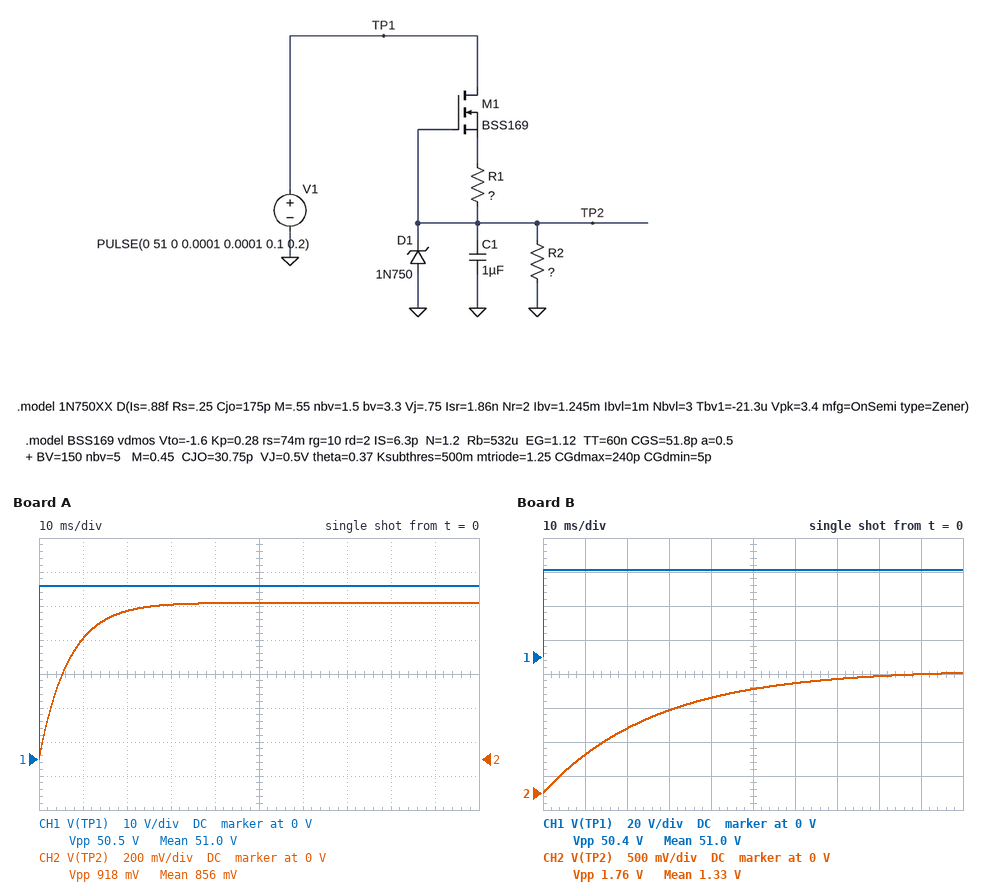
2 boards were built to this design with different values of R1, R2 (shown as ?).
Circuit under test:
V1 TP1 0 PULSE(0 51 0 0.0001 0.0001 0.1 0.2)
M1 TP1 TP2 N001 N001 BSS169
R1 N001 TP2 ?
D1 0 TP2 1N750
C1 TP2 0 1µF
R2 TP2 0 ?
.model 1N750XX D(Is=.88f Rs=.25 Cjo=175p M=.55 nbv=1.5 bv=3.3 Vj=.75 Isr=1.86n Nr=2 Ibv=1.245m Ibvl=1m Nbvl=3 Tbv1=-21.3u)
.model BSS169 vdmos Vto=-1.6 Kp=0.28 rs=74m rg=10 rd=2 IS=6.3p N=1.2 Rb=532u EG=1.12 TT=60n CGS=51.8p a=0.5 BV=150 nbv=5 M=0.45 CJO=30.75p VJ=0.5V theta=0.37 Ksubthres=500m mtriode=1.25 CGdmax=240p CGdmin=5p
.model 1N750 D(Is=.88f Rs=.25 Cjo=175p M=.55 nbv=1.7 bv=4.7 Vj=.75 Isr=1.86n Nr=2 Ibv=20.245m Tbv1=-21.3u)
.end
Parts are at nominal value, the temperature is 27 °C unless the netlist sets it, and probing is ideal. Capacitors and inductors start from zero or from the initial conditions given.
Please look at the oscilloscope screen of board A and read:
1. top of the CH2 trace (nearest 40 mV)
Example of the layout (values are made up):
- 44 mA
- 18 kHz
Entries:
- 920 mV
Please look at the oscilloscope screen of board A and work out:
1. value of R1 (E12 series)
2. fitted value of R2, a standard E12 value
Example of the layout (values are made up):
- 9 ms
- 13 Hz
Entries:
- 22 kΩ
- 6.8 kΩ
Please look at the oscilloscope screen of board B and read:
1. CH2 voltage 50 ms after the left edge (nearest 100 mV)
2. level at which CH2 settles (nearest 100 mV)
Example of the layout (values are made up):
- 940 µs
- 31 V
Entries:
- 1.5 V
- 1.8 V
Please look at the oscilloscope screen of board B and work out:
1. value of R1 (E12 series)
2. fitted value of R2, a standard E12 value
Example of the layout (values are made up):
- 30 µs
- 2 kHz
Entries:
- 47 kΩ
- 27 kΩ
